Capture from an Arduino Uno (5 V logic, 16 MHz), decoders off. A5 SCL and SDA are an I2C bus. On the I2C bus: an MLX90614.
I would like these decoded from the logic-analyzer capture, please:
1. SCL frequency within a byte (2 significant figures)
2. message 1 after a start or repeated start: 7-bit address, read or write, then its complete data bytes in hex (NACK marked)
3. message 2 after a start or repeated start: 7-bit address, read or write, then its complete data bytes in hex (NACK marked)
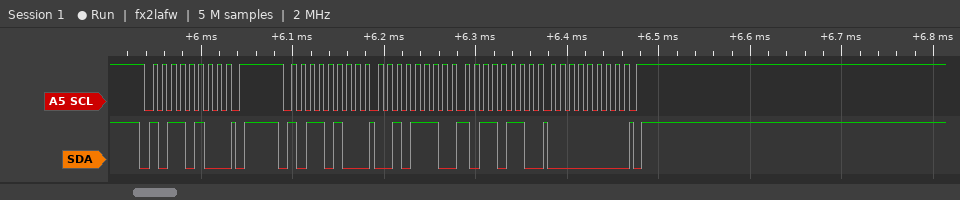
100 kHz
0x5A write
0x5A write: 2E B6 00
